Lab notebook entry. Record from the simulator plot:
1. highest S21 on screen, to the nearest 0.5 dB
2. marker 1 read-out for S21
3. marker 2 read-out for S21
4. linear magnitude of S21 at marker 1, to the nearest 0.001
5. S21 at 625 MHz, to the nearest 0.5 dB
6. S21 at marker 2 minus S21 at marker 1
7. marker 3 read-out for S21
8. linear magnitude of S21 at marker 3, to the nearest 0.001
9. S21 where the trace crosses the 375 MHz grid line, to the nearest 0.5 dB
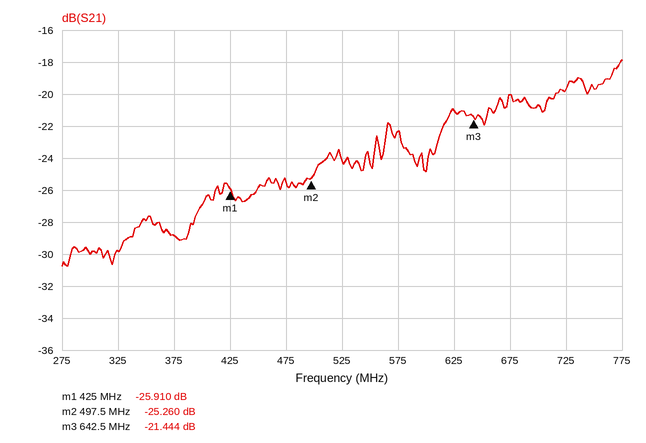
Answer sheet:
-18.0 dB
-25.910 dB
-25.260 dB
0.051
-21.0 dB
0.650 dB
-21.444 dB
0.085
-29.0 dB
